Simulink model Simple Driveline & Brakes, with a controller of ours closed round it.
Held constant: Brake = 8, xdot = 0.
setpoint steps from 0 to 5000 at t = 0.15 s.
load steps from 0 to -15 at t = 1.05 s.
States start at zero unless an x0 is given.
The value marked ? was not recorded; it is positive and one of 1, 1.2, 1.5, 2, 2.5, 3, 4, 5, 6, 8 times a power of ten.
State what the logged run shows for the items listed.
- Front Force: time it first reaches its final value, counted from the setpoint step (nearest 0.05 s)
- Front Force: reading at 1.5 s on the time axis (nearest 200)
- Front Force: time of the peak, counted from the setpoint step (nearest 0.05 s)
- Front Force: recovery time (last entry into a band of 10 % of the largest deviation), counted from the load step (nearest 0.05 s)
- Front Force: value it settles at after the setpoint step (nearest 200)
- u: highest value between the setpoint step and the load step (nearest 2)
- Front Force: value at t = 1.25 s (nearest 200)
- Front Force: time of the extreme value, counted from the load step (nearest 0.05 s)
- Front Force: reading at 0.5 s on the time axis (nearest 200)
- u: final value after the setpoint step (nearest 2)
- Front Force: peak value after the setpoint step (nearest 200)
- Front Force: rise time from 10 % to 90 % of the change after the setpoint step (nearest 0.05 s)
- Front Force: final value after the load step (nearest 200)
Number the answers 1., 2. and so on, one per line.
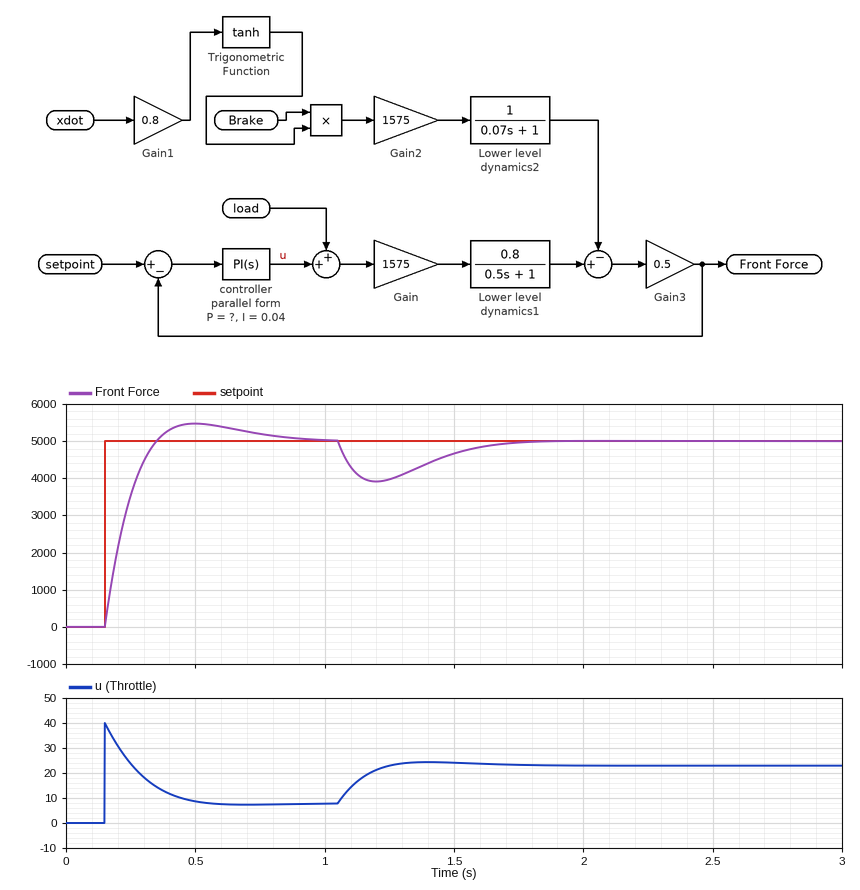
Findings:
1. 0.20 s
2. 4600
3. 0.35 s
4. 0.60 s
5. 5000
6. 40
7. 4000
8. 0.15 s
9. 5400
10. 8
11. 5400
12. 0.15 s
13. 5000
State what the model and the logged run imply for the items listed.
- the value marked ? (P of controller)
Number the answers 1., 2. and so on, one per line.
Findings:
1. 0.008
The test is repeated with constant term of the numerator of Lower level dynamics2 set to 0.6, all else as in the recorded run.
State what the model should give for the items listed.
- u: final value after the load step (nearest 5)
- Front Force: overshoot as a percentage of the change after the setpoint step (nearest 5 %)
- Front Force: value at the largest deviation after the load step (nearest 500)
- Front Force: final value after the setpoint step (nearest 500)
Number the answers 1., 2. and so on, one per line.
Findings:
1. 25
2. 10 %
3. 4000
4. 5000
